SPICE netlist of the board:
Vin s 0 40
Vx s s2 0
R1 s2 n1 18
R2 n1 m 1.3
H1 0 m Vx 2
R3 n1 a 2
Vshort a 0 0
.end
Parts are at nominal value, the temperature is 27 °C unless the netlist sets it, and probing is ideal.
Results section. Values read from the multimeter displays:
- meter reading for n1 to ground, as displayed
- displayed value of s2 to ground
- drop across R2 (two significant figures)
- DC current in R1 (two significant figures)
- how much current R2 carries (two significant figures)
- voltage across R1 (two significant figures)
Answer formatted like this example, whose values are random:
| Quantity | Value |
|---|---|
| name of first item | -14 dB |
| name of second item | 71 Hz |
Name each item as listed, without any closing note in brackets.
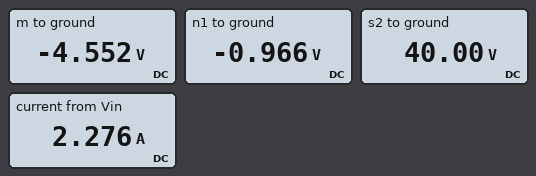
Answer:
| Quantity | Value |
|---|---|
| meter reading for n1 to ground, as displayed | -0.966 V |
| displayed value of s2 to ground | 40.00 V |
| drop across R2 | 3.6 V |
| DC current in R1 | 2.3 A |
| how much current R2 carries | 2.8 A |
| voltage across R1 | 41 V |
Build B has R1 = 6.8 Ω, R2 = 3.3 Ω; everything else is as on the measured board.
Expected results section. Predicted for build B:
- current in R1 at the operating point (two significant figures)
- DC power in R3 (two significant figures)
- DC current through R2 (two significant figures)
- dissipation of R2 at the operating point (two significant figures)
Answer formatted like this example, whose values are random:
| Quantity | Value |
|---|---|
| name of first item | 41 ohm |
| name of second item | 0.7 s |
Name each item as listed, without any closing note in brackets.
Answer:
| Quantity | Value |
|---|---|
| current in R1 at the operating point | 5.5 A |
| DC power in R3 | 3.6 W |
| DC current through R2 | 4.1 A |
| dissipation of R2 at the operating point | 57 W |
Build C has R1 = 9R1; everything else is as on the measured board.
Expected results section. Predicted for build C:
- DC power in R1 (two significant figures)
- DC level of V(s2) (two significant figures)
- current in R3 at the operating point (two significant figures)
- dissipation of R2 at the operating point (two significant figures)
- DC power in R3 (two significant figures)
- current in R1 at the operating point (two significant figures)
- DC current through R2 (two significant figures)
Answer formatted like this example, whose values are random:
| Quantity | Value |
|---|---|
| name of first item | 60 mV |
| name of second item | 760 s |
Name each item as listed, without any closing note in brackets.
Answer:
| Quantity | Value |
|---|---|
| DC power in R1 | 190 W |
| DC level of V(s2) | 40 V |
| current in R3 at the operating point | 980 mA |
| dissipation of R2 at the operating point | 41 W |
| DC power in R3 | 1.9 W |
| current in R1 at the operating point | 4.6 A |
| DC current through R2 | 5.6 A |
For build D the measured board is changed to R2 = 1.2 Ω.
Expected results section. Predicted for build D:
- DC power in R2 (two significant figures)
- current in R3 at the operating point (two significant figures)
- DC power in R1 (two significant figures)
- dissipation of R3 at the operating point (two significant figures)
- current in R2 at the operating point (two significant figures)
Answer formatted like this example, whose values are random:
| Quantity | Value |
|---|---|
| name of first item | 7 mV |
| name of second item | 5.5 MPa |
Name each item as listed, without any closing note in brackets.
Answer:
| Quantity | Value |
|---|---|
| DC power in R2 | 9.8 W |
| current in R3 at the operating point | 570 mA |
| DC power in R1 | 94 W |
| dissipation of R3 at the operating point | 650 mW |
| current in R2 at the operating point | 2.9 A |
